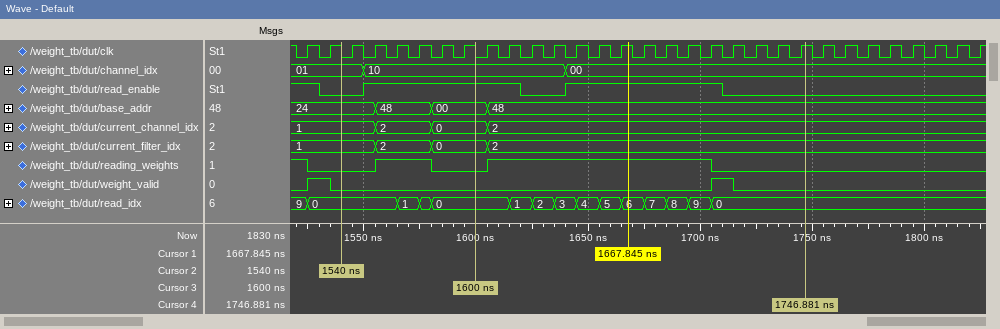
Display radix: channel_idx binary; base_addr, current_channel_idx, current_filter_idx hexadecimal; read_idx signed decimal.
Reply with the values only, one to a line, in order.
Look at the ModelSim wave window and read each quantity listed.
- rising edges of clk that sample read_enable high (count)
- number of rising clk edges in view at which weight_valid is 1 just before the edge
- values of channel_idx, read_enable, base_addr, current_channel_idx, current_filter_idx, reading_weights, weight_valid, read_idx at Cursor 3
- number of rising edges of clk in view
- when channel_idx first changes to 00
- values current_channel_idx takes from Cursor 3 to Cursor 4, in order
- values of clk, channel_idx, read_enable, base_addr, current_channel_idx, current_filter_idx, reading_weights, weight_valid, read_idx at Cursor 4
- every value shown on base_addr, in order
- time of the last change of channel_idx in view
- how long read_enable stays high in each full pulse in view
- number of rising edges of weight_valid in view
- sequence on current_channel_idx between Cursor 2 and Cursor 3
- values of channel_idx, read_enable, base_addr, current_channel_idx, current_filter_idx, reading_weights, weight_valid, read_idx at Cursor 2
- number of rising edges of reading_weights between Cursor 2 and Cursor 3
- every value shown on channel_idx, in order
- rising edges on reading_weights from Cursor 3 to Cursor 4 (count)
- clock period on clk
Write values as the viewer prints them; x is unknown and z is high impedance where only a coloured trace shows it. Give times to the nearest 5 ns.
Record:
15
2
channel_idx=10, read_enable=1, base_addr=00, current_channel_idx=0, current_filter_idx=0, reading_weights=0, weight_valid=0, read_idx=0
31
1640 ns
0, 2
clk=1, channel_idx=00, read_enable=0, base_addr=48, current_channel_idx=2, current_filter_idx=2, reading_weights=0, weight_valid=0, read_idx=0
24, 48, 00, 48
1640 ns
70 ns, 70 ns
2
1, 2, 0
channel_idx=01, read_enable=0, base_addr=24, current_channel_idx=1, current_filter_idx=1, reading_weights=0, weight_valid=0, read_idx=0
1
01, 10, 00
1
10 ns
